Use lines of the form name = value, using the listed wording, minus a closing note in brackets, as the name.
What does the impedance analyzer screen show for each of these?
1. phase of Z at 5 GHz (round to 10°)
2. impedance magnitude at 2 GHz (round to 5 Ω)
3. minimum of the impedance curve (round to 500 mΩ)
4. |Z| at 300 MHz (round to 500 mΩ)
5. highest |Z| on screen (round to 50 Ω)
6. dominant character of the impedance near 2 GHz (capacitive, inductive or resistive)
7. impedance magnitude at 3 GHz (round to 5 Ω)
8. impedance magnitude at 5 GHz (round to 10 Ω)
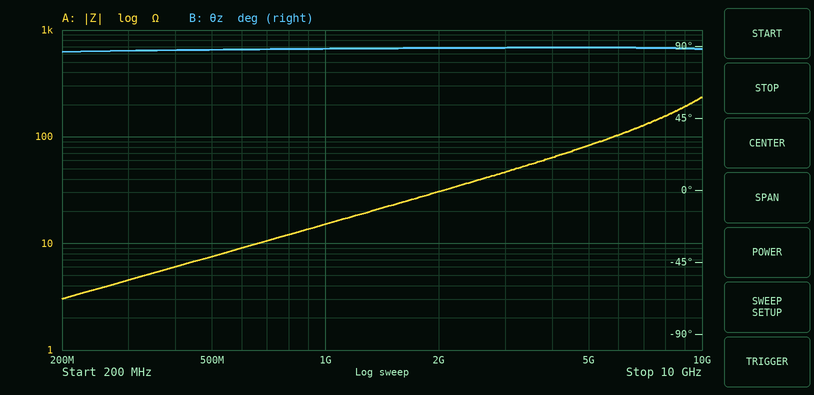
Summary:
phase of Z at 5 GHz = 90°
impedance magnitude at 2 GHz = 30 Ω
minimum of the impedance curve = 3.0 Ω
|Z| at 300 MHz = 4.5 Ω
highest |Z| on screen = 250 Ω
dominant character of the impedance near 2 GHz = inductive
impedance magnitude at 3 GHz = 45 Ω
impedance magnitude at 5 GHz = 80 Ω
